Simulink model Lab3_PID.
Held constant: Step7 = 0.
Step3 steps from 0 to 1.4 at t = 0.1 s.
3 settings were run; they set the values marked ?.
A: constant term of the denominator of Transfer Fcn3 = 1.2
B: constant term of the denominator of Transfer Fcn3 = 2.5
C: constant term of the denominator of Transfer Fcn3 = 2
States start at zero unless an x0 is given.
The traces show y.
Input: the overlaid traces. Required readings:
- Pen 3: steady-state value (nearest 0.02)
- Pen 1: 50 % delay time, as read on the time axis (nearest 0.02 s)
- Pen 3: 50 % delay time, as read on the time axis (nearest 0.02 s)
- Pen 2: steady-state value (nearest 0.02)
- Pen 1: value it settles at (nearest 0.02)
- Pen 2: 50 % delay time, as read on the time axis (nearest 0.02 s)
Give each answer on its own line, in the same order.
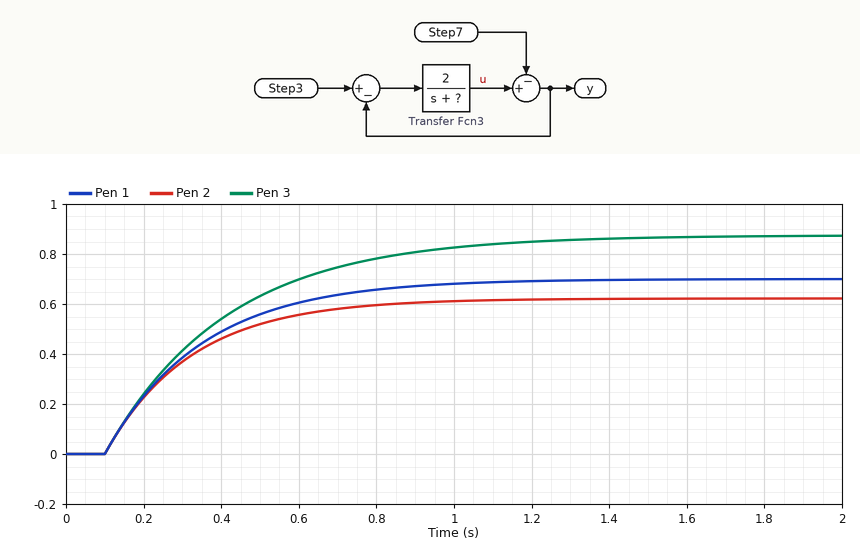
0.88
0.28 s
0.32 s
0.62
0.70
0.26 s
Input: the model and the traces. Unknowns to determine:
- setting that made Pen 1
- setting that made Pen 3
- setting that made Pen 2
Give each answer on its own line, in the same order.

C
A
B
